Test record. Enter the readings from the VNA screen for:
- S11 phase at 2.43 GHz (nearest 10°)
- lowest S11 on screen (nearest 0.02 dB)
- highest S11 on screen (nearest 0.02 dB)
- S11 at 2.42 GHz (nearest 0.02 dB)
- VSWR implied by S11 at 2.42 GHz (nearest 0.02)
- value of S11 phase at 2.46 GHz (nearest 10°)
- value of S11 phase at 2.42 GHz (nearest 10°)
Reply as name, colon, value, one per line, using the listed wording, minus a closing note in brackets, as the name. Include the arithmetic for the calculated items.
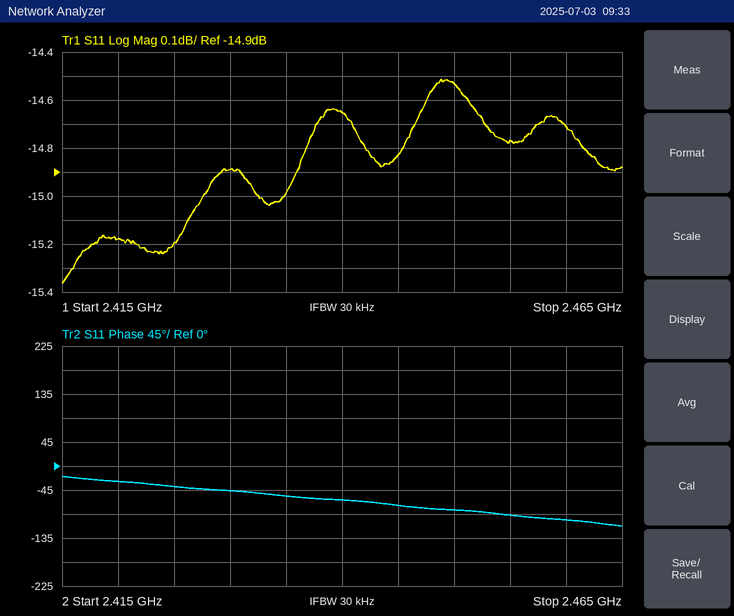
S11 phase at 2.43 GHz: -50°
lowest S11 on screen: -15.36 dB
highest S11 on screen: -14.52 dB
S11 at 2.42 GHz: -15.18 dB
VSWR implied by S11 at 2.42 GHz: |Γ| = 10^(-15.18/20) = 0.1742; VSWR = (1 + 0.1742)/(1 − 0.1742) ≈ 1.42
value of S11 phase at 2.46 GHz: -100°
value of S11 phase at 2.42 GHz: -30°
